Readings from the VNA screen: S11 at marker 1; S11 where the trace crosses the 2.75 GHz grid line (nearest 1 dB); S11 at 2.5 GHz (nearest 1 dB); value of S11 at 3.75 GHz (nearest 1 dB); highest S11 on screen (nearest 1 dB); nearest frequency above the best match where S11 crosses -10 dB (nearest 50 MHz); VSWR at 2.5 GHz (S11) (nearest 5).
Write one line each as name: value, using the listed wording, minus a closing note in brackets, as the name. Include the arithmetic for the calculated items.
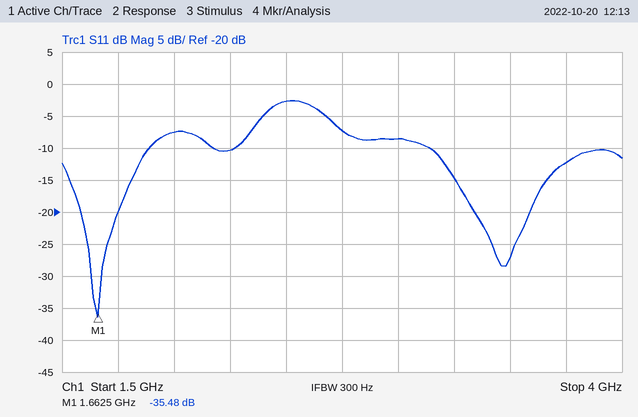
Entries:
S11 at marker 1: -35.48 dB
S11 where the trace crosses the 2.75 GHz grid line: -7 dB
S11 at 2.5 GHz: -3 dB
value of S11 at 3.75 GHz: -12 dB
highest S11 on screen: -3 dB
nearest frequency above the best match where S11 crosses -10 dB: 1.90 GHz
VSWR at 2.5 GHz (S11): |Γ| = 10^(-3/20) = 0.7079; VSWR = (1 + 0.7079)/(1 − 0.7079) ≈ 5.85, so 5 to the nearest 5
